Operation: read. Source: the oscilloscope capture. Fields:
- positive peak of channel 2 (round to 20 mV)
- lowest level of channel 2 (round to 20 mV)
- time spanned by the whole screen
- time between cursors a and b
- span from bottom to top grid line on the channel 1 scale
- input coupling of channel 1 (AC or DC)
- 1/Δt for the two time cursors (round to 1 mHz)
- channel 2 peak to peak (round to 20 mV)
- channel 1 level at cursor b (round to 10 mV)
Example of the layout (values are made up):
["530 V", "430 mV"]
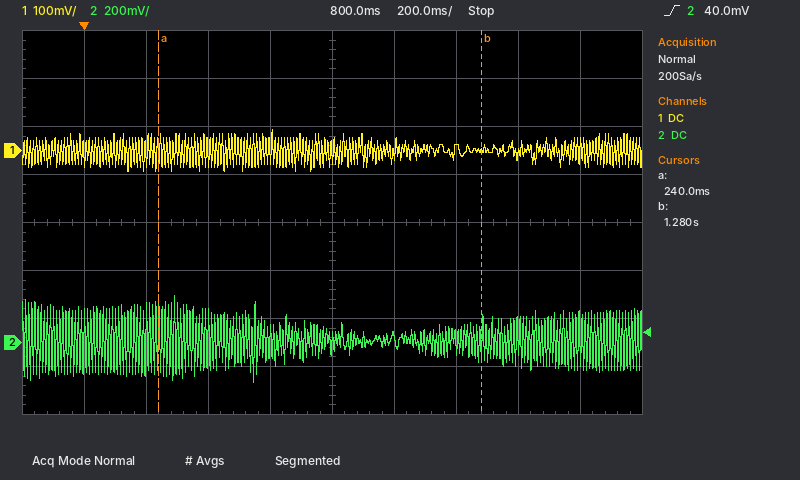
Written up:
["200 mV", "-160 mV", "2 s", "1.04 s", "800 mV", "DC", "962 mHz", "360 mV", "0 mV"]
